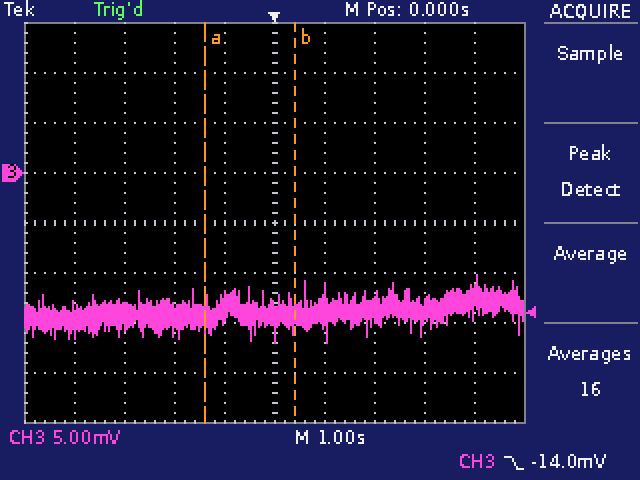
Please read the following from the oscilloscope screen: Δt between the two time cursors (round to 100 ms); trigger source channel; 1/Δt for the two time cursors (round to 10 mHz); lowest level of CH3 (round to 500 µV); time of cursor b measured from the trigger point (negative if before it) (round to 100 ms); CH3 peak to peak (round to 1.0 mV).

1.8 s
CH3
560 mHz
-17.0 mV
+400 ms
7.0 mV
